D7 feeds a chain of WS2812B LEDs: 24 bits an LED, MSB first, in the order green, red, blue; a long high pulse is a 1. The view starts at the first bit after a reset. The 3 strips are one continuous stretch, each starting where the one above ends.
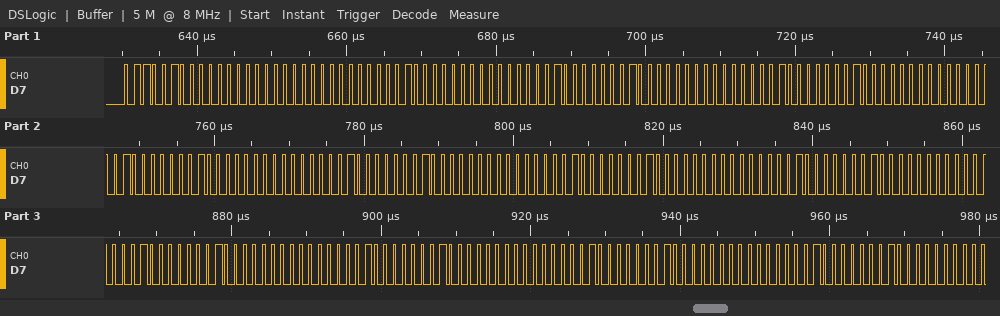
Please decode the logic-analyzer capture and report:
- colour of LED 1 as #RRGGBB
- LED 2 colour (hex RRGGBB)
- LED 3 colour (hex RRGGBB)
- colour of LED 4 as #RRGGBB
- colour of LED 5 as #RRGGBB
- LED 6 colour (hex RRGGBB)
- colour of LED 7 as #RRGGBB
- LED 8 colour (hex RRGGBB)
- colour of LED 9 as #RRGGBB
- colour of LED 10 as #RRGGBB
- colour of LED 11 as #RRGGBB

#006400
#000202
#000202
#000202
#000202
#000202
#000202
#000202
#000202
#000202
#000202
